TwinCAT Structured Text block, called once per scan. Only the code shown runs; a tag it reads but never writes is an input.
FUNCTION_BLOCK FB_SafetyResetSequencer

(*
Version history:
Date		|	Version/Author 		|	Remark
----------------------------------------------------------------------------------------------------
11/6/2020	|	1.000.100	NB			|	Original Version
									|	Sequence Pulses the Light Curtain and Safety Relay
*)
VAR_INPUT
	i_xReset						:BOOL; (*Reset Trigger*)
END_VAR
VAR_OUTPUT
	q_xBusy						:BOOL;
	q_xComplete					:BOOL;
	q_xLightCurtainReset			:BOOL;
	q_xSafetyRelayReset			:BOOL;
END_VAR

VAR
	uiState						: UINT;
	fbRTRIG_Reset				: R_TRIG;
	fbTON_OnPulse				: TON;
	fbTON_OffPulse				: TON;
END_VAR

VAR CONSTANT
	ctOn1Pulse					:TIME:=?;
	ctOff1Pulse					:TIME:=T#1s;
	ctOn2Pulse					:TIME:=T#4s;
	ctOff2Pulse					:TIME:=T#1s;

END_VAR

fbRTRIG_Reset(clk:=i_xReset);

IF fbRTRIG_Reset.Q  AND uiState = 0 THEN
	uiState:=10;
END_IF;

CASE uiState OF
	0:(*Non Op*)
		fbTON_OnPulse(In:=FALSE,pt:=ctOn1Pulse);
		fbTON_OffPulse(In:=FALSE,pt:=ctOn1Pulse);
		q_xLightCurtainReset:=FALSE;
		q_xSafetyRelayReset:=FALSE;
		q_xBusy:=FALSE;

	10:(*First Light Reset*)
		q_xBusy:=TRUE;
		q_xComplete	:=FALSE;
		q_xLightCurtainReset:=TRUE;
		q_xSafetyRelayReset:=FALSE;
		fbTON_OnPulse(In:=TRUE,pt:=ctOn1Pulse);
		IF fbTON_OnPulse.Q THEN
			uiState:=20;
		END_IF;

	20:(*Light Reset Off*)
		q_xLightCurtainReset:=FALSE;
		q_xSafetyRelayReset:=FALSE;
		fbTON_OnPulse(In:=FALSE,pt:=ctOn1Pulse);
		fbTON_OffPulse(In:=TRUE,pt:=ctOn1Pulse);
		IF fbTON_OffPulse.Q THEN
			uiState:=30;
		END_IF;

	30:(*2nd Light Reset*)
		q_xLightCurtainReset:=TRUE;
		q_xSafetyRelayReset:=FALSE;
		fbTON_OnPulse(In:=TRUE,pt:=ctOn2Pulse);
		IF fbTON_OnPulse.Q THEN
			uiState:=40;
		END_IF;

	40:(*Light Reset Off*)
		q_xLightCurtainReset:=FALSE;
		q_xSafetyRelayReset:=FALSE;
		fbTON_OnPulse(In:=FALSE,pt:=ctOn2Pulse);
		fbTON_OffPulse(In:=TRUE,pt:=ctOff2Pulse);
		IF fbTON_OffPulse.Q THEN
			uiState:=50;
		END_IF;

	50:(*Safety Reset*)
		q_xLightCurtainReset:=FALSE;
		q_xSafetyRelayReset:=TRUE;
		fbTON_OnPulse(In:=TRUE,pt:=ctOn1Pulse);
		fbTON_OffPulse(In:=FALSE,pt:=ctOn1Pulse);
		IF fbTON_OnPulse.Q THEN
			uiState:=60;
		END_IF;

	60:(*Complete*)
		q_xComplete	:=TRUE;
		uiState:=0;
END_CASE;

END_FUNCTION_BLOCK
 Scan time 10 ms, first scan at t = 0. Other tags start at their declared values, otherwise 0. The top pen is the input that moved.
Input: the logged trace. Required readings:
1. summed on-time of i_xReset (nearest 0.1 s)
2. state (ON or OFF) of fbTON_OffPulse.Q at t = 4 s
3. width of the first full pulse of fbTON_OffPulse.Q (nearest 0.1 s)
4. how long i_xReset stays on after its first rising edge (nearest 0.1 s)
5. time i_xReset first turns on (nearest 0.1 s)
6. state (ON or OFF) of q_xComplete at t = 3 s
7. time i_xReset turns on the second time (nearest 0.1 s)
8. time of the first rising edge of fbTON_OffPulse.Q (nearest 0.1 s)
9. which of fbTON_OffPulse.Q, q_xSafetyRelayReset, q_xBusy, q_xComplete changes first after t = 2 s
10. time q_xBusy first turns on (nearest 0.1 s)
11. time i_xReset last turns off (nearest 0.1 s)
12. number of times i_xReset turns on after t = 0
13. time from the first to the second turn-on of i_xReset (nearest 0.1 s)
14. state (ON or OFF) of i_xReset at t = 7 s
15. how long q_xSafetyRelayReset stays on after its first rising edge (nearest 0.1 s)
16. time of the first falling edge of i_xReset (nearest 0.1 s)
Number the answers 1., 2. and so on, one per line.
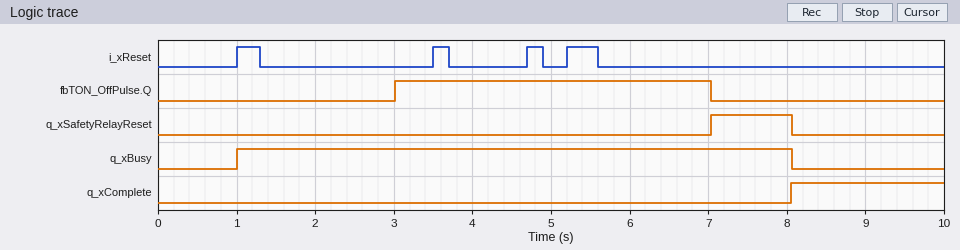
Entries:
1. 1.1 s
2. ON
3. 4.0 s
4. 0.3 s
5. 1.0 s
6. OFF
7. 3.5 s
8. 3.0 s
9. fbTON_OffPulse.Q
10. 1.0 s
11. 5.6 s
12. 4
13. 2.5 s
14. OFF
15. 1.0 s
16. 1.3 s
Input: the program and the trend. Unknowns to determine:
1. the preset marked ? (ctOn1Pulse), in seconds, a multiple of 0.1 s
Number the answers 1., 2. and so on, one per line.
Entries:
1. 1.0 s
